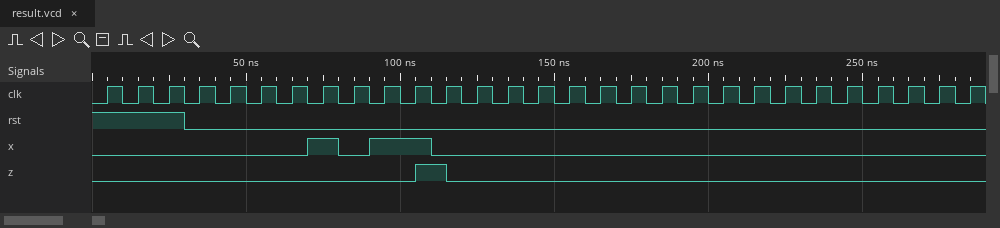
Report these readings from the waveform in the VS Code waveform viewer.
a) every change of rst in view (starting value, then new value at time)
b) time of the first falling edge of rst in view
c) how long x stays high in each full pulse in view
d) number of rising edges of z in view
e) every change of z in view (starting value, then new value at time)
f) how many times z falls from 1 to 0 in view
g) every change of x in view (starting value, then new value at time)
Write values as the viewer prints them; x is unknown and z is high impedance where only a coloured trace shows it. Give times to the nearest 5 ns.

1, 0 at 30 ns
30 ns
10 ns, 20 ns
1
0, 1 at 105 ns, 0 at 115 ns
1
0, 1 at 70 ns, 0 at 80 ns, 1 at 90 ns, 0 at 110 ns
